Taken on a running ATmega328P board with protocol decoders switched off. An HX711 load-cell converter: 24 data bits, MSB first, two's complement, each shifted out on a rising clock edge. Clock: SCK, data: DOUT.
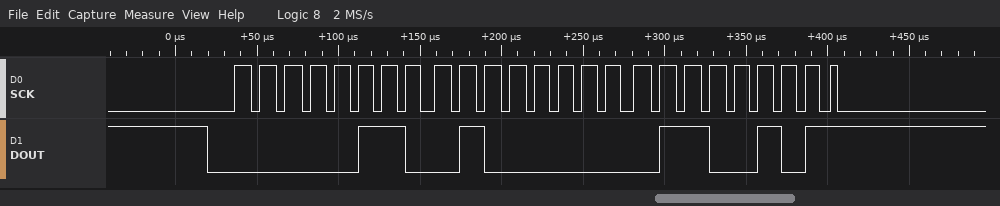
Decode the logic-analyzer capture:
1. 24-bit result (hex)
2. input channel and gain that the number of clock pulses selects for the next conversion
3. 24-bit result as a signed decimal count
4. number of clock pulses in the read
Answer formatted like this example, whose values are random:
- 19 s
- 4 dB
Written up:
- 0x064065
- channel A, gain 128
- 409701
- 25
